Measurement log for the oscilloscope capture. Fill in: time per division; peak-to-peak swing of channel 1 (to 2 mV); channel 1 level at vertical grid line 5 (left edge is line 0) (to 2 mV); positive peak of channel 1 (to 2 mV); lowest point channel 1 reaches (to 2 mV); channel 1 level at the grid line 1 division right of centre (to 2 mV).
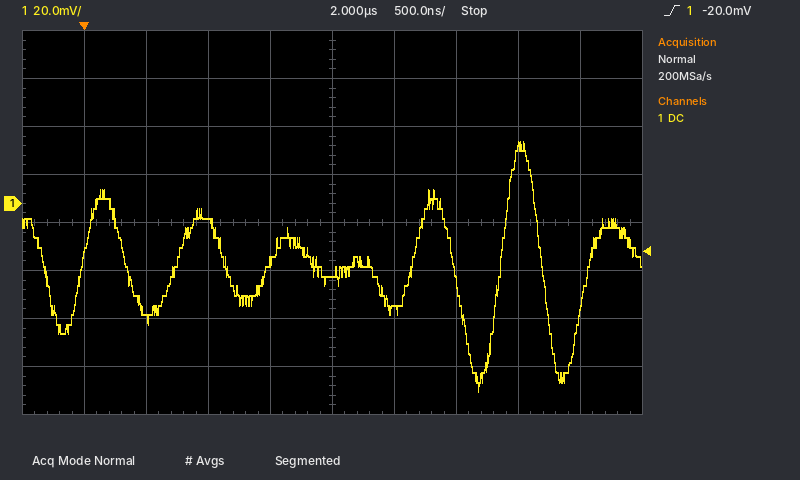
500 ns
104 mV
-30 mV
26 mV
-78 mV
-44 mV
